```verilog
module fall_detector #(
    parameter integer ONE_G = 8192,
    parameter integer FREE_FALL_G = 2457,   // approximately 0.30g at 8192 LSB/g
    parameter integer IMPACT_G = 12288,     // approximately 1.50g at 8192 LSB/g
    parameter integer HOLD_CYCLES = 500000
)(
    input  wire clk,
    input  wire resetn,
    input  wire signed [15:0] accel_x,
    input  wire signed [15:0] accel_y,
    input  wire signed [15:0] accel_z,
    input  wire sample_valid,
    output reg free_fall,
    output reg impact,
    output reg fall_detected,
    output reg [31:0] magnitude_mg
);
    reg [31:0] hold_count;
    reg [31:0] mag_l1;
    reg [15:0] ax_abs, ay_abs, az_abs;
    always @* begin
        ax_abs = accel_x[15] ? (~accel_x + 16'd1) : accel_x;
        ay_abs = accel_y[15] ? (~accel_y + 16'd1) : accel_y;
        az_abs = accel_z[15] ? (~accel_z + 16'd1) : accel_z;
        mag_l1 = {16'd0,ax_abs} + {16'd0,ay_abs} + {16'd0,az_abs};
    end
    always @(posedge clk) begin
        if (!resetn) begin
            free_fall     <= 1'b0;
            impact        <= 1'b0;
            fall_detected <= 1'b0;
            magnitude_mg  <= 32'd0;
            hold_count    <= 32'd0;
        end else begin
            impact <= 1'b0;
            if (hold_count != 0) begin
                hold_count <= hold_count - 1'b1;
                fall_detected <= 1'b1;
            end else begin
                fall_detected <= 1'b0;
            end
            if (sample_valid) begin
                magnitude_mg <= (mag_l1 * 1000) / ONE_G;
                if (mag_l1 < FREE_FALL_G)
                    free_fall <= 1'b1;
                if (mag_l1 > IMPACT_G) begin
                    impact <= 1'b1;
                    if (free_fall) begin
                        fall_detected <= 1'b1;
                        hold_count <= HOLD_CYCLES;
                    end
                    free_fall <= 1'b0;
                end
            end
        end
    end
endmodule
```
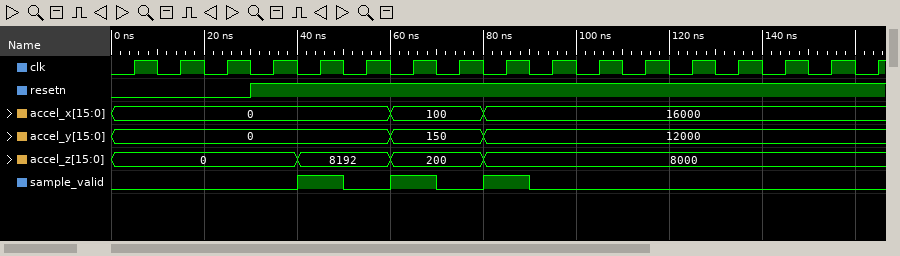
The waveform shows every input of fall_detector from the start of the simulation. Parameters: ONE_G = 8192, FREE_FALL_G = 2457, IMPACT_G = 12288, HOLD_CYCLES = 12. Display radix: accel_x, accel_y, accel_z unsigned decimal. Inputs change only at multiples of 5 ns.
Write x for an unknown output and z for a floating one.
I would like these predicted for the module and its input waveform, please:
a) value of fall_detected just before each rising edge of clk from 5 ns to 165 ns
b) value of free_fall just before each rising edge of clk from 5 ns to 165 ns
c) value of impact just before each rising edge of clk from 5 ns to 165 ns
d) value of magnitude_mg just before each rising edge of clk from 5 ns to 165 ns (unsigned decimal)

x 0 0 0 0 0 0 0 0 1 1 1 1 1 1 1 1
x 0 0 0 0 0 0 1 1 0 0 0 0 0 0 0 0
x 0 0 0 0 0 0 0 0 1 0 0 0 0 0 0 0
x, 0, 0, 0, 0, 1000, 1000, 54, 54, 4394, 4394, 4394, 4394, 4394, 4394, 4394, 4394
